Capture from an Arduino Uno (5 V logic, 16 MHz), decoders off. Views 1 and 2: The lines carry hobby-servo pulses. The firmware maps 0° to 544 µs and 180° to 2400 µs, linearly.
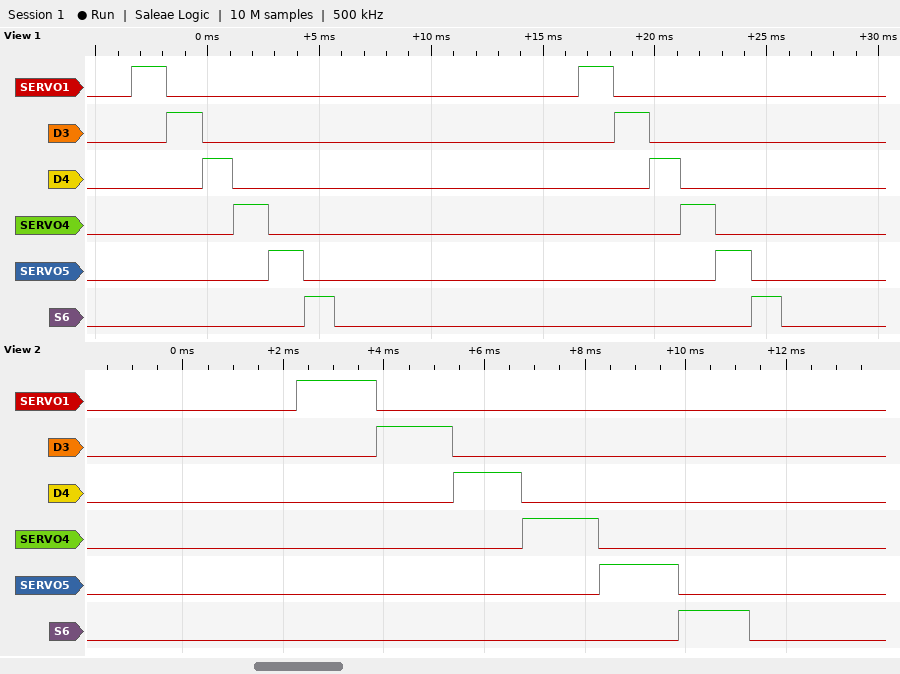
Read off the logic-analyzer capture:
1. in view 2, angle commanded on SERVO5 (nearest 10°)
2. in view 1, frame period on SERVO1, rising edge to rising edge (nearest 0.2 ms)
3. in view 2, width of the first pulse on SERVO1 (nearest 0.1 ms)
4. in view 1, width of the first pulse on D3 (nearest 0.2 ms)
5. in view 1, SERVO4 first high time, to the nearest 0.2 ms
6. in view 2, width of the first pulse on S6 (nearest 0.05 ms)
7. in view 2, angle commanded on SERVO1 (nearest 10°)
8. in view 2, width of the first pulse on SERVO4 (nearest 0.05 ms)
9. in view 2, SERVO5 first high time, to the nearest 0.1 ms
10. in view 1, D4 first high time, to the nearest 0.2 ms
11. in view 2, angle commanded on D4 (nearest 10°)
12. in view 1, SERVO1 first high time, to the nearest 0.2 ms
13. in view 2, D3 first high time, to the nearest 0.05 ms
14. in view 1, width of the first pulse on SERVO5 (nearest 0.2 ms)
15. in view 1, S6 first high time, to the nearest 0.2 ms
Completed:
100°
20.0 ms
1.6 ms
1.6 ms
1.6 ms
1.40 ms
100°
1.50 ms
1.6 ms
1.4 ms
80°
1.6 ms
1.50 ms
1.6 ms
1.4 ms
